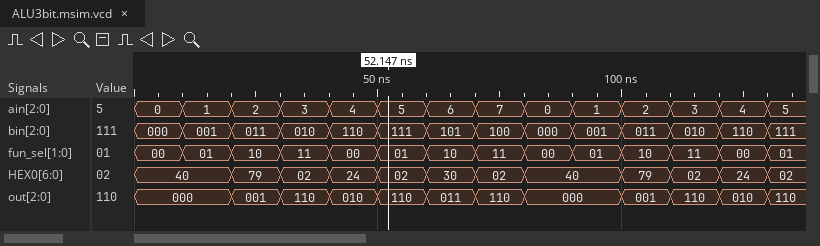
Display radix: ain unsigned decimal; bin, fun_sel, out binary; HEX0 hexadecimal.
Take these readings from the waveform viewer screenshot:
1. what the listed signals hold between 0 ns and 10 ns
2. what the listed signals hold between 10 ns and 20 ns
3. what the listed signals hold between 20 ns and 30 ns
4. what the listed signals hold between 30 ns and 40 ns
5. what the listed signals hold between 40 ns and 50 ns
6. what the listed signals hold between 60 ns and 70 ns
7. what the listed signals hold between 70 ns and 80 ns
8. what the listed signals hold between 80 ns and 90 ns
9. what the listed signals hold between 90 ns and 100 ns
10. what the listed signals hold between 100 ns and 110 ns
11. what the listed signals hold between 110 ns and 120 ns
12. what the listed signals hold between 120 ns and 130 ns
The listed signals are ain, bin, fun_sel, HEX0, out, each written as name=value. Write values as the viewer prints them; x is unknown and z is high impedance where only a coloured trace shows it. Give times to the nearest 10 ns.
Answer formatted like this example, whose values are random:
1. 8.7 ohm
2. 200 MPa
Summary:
1. ain=0, bin=000, fun_sel=00, HEX0=40, out=000
2. ain=1, bin=001, fun_sel=01, HEX0=40, out=000
3. ain=2, bin=011, fun_sel=10, HEX0=79, out=001
4. ain=3, bin=010, fun_sel=11, HEX0=02, out=110
5. ain=4, bin=110, fun_sel=00, HEX0=24, out=010
6. ain=6, bin=101, fun_sel=10, HEX0=30, out=011
7. ain=7, bin=100, fun_sel=11, HEX0=02, out=110
8. ain=0, bin=000, fun_sel=00, HEX0=40, out=000
9. ain=1, bin=001, fun_sel=01, HEX0=40, out=000
10. ain=2, bin=011, fun_sel=10, HEX0=79, out=001
11. ain=3, bin=010, fun_sel=11, HEX0=02, out=110
12. ain=4, bin=110, fun_sel=00, HEX0=24, out=010
